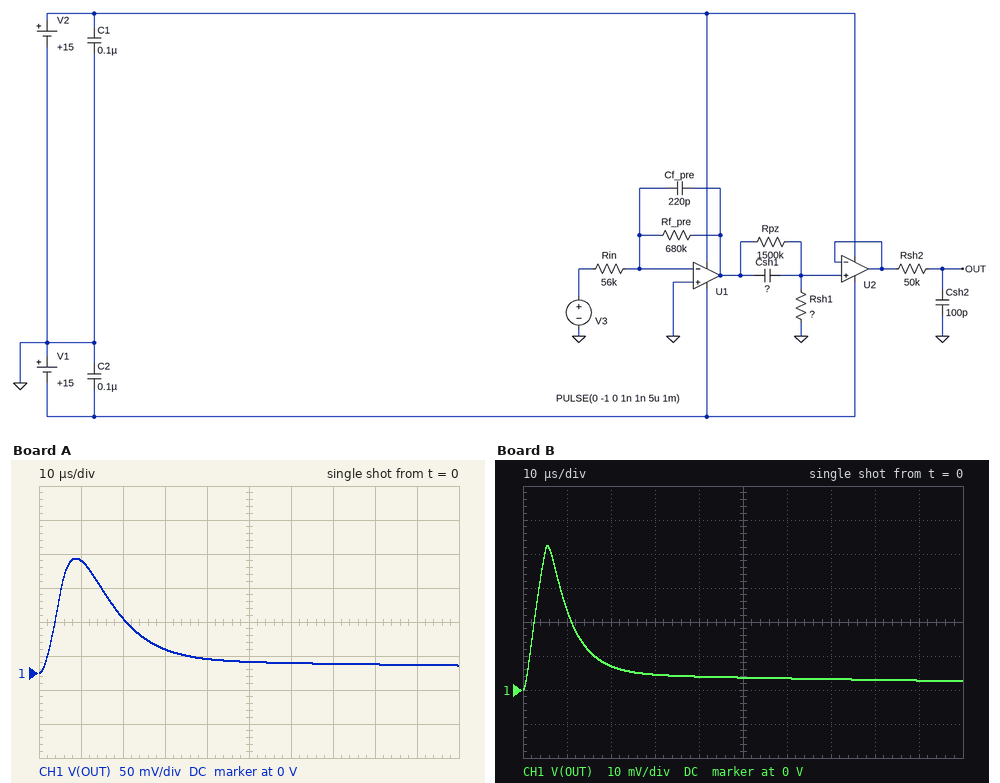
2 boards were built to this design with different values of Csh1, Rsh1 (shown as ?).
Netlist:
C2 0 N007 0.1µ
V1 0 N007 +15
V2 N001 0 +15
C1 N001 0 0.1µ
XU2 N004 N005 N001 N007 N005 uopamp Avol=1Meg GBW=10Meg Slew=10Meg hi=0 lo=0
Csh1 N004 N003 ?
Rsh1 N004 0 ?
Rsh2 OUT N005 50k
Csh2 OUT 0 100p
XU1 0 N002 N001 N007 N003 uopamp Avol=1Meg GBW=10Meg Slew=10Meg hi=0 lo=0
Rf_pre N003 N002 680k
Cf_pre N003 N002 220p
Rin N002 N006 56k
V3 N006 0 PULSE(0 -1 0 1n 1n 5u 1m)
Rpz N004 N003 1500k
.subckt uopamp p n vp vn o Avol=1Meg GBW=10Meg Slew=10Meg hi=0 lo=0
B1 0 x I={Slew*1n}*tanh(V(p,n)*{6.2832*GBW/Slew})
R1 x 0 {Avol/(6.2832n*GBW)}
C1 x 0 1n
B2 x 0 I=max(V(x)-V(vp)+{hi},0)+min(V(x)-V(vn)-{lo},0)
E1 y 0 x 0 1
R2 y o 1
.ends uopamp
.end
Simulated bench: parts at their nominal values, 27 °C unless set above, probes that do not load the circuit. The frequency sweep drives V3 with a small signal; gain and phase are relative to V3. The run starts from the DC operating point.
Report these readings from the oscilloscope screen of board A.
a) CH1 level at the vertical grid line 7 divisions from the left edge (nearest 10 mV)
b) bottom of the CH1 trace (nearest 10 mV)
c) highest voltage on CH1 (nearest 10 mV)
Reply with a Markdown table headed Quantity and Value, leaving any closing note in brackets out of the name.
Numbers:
| Quantity | Value |
|---|---|
| CH1 level at the vertical grid line 7 divisions from the left edge | 10 mV |
| bottom of the CH1 trace | 0 V |
| highest voltage on CH1 | 170 mV |
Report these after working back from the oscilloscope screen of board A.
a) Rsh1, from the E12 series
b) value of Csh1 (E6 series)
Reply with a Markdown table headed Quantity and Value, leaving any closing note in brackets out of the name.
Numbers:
| Quantity | Value |
|---|---|
| Rsh1, from the E12 series | 150 kΩ |
| value of Csh1 | 47 pF |
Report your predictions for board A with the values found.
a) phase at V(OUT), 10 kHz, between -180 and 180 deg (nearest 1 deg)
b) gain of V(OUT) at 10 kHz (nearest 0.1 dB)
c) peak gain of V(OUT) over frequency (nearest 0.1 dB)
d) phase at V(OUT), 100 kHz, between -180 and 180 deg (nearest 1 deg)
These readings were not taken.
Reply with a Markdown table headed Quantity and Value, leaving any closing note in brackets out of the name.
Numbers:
| Quantity | Value |
|---|---|
| phase at V(OUT), 10 kHz, between -180 and 180 deg | 134 deg |
| gain of V(OUT) at 10 kHz | -6.6 dB |
| peak gain of V(OUT) over frequency | 0.9 dB |
| phase at V(OUT), 100 kHz, between -180 and 180 deg | 30 deg |
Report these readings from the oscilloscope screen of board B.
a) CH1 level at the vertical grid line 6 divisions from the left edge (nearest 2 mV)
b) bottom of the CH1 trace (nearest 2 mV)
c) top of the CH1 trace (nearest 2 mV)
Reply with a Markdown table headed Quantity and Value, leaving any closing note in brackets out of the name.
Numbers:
| Quantity | Value |
|---|---|
| CH1 level at the vertical grid line 6 divisions from the left edge | 4 mV |
| bottom of the CH1 trace | 0 V |
| top of the CH1 trace | 42 mV |
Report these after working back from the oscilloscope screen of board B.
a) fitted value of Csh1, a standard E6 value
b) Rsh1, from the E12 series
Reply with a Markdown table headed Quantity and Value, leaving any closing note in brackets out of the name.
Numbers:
| Quantity | Value |
|---|---|
| fitted value of Csh1, a standard E6 value | 33 pF |
| Rsh1, from the E12 series | 27 kΩ |
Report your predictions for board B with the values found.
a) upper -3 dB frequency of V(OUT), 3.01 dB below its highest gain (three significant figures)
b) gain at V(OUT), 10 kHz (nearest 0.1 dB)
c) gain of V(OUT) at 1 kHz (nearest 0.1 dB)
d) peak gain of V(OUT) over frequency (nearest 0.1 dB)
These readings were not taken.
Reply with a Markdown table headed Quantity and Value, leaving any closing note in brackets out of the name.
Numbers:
| Quantity | Value |
|---|---|
| upper -3 dB frequency of V(OUT), 3.01 dB below its highest gain | 1.20 kHz |
| gain at V(OUT), 10 kHz | -23.0 dB |
| gain of V(OUT) at 1 kHz | -15.7 dB |
| peak gain of V(OUT) over frequency | -13.4 dB |
